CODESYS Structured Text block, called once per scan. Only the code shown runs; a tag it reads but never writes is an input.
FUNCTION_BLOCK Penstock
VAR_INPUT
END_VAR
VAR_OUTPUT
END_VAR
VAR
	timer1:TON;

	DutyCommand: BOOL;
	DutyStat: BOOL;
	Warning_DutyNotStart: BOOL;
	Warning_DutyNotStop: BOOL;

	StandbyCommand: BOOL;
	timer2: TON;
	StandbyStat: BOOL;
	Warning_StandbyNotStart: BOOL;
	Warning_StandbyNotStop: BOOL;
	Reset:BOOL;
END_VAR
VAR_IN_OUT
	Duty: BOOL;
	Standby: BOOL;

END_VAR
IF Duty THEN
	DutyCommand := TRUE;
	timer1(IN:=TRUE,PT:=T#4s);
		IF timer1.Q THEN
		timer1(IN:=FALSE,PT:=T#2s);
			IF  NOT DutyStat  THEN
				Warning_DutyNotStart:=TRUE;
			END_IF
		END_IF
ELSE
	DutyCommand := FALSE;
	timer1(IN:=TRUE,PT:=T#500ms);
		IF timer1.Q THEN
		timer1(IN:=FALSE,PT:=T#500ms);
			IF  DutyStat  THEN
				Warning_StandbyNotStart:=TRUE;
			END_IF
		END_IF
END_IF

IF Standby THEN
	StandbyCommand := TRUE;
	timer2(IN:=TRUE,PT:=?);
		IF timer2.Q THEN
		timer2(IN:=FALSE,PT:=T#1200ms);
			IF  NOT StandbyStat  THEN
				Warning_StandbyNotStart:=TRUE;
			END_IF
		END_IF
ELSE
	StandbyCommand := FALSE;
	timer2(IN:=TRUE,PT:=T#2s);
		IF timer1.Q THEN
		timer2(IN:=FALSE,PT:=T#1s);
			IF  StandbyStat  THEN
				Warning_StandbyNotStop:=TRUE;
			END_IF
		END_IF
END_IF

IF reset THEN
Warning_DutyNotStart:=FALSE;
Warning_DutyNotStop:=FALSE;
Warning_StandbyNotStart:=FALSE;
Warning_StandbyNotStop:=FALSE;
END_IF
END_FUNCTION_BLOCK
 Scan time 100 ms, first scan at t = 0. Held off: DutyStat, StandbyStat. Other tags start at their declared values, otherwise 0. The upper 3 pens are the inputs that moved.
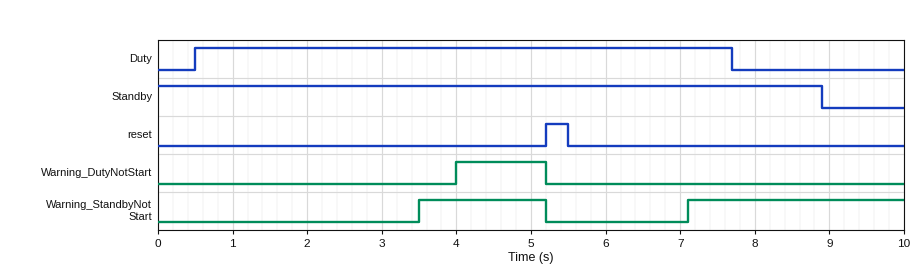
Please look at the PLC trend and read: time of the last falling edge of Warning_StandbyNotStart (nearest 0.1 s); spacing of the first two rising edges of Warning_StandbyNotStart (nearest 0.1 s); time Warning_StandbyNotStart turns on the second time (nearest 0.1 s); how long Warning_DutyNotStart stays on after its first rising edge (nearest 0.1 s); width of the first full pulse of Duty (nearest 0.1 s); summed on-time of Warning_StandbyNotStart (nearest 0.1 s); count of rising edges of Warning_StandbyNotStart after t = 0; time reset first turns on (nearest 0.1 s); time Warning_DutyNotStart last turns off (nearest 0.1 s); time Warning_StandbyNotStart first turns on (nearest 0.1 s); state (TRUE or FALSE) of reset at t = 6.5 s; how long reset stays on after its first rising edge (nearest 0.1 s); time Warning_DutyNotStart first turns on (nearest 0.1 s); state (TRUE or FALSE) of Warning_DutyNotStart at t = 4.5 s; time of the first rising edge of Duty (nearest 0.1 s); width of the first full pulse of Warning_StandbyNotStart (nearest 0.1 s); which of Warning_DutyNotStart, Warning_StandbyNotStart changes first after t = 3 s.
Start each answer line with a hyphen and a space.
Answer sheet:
- 5.2 s
- 3.6 s
- 7.1 s
- 1.2 s
- 7.2 s
- 4.6 s
- 2
- 5.2 s
- 5.2 s
- 3.5 s
- FALSE
- 0.3 s
- 4.0 s
- TRUE
- 0.5 s
- 1.7 s
- Warning_StandbyNotStart
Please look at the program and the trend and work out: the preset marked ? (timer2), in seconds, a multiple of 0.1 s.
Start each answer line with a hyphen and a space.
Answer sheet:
- 3.5 s
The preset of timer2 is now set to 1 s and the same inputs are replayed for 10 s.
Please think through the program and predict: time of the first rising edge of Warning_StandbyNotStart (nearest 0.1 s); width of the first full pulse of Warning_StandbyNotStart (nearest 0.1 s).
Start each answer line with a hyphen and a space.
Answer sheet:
- 1.0 s
- 4.2 s
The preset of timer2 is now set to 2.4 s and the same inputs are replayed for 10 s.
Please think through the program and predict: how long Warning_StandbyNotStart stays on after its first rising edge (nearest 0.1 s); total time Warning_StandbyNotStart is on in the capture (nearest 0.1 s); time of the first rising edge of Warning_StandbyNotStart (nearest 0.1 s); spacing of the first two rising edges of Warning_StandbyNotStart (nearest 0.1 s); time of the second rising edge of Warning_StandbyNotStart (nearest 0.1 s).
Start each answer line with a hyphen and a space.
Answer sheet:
- 2.8 s
- 5.4 s
- 2.4 s
- 5.0 s
- 7.4 s
